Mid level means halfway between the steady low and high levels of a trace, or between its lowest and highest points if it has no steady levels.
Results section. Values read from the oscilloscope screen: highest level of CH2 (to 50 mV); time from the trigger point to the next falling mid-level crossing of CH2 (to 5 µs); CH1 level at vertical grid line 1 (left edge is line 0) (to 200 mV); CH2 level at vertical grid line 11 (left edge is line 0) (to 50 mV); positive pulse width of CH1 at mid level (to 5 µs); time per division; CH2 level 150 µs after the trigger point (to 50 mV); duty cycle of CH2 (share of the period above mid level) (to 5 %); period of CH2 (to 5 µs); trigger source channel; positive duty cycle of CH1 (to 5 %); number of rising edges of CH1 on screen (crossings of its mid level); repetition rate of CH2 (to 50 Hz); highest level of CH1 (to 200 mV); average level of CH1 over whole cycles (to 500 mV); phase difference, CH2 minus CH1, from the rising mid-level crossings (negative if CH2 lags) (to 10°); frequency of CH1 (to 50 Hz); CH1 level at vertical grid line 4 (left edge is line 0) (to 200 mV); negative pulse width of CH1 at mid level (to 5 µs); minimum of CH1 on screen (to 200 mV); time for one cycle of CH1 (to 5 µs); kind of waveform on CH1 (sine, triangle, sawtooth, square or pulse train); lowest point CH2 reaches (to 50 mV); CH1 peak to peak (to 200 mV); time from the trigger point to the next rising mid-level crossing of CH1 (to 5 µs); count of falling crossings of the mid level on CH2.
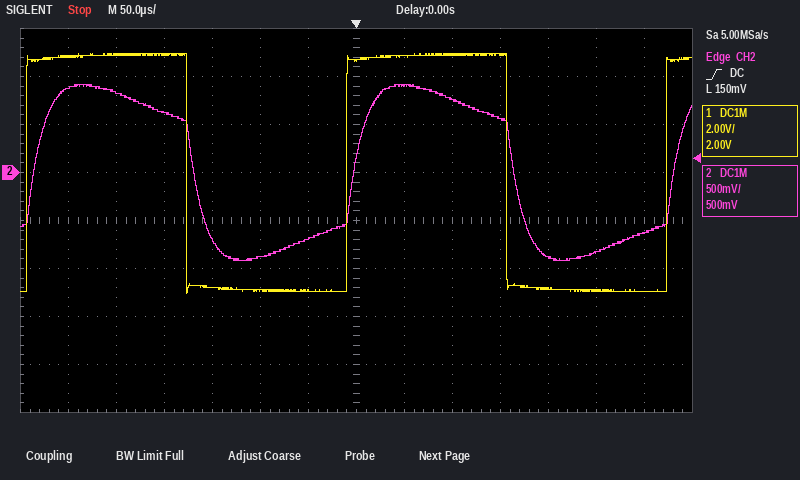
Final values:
900 mV
165 µs
4.8 V
-900 mV
165 µs
50 µs
550 mV
50 %
335 µs
CH2
50 %
3
3.00 kHz
5.0 V
0.0 V
-10°
3.00 kHz
-4.8 V
165 µs
-5.0 V
335 µs
square
-900 mV
10.0 V
325 µs
2
